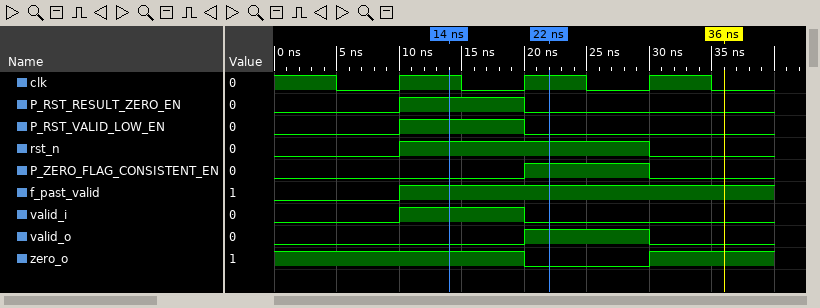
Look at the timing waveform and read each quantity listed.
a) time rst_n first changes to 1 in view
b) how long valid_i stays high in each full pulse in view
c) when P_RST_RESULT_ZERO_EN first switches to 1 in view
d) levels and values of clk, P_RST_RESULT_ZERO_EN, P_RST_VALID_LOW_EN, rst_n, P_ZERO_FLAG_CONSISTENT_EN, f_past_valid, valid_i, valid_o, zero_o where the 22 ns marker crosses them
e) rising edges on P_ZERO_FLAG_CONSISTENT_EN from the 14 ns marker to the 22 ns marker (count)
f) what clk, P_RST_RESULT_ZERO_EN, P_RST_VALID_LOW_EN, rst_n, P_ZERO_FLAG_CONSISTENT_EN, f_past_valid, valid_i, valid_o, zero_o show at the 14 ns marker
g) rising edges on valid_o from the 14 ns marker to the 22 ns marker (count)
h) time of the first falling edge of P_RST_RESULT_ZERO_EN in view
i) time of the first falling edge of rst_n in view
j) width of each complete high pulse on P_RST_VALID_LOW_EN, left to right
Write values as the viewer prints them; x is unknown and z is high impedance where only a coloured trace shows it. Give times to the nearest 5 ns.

10 ns
10 ns
10 ns
clk=1, P_RST_RESULT_ZERO_EN=0, P_RST_VALID_LOW_EN=0, rst_n=1, P_ZERO_FLAG_CONSISTENT_EN=1, f_past_valid=1, valid_i=0, valid_o=1, zero_o=0
1
clk=1, P_RST_RESULT_ZERO_EN=1, P_RST_VALID_LOW_EN=1, rst_n=1, P_ZERO_FLAG_CONSISTENT_EN=0, f_past_valid=1, valid_i=1, valid_o=0, zero_o=1
1
20 ns
30 ns
10 ns
